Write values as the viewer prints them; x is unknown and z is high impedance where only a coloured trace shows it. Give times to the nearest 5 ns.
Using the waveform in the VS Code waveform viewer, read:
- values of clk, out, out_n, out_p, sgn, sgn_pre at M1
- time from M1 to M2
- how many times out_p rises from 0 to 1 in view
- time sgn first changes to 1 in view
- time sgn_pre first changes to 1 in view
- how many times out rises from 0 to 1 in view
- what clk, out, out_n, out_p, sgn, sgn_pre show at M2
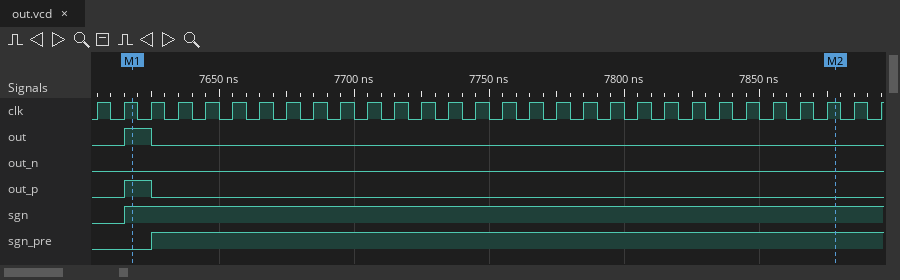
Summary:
clk=1, out=1, out_n=0, out_p=1, sgn=1, sgn_pre=0
260 ns
1
7615 ns
7625 ns
1
clk=1, out=0, out_n=0, out_p=0, sgn=1, sgn_pre=1
